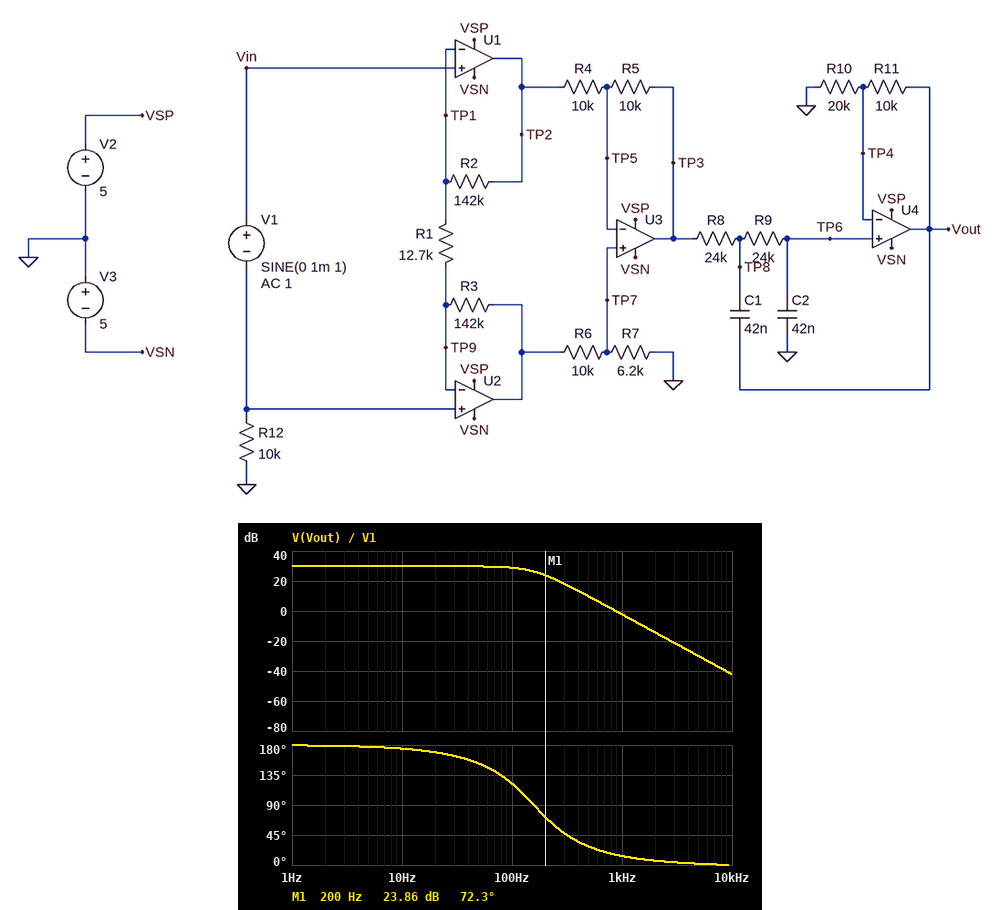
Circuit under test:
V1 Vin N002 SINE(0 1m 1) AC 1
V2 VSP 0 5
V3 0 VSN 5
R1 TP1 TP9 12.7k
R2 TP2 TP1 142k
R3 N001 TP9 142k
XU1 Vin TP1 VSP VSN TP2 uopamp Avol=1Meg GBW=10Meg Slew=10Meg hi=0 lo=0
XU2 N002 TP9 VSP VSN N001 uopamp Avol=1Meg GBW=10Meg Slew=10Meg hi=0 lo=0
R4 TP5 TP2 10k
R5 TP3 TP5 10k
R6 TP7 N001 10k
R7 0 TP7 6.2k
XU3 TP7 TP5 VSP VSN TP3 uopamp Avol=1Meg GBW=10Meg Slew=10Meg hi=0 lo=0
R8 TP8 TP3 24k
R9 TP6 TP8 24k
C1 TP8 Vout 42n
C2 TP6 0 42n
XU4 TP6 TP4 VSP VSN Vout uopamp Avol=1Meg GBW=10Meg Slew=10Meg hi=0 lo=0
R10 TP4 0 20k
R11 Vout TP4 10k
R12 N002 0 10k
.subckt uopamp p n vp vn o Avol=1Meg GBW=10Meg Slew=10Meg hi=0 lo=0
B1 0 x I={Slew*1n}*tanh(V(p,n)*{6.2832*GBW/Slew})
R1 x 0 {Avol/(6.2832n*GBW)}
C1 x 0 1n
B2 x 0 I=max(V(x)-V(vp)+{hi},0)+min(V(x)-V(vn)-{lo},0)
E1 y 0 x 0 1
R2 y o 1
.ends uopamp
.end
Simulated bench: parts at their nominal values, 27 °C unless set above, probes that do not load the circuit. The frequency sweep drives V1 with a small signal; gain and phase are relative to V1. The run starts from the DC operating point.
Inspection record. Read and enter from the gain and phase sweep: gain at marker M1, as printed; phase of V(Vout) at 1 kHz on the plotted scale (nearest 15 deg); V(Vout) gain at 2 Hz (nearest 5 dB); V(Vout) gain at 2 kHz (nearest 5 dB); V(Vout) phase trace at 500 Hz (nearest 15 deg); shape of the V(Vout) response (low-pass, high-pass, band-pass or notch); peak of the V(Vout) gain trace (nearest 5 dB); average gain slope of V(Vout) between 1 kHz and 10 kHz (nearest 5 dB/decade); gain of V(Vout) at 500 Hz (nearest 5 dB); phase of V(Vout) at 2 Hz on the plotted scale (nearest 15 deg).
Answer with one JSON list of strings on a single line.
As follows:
["23.86 dB", "15 deg", "30 dB", "-15 dB", "30 deg", "low-pass", "30 dB", "-40 dB/decade", "10 dB", "180 deg"]
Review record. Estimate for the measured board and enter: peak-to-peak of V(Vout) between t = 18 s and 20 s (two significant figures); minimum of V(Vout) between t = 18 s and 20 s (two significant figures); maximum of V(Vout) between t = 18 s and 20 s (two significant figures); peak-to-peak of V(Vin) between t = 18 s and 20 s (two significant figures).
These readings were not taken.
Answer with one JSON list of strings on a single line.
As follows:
["62 mV", "-31 mV", "31 mV", "2.0 mV"]
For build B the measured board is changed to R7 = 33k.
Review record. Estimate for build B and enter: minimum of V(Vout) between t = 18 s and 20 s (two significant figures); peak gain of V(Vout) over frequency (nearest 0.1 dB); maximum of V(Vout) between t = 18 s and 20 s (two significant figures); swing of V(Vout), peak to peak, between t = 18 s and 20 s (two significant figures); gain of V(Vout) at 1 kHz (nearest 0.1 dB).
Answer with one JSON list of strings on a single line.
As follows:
["-44 mV", "32.9 dB", "44 mV", "88 mV", "0.8 dB"]
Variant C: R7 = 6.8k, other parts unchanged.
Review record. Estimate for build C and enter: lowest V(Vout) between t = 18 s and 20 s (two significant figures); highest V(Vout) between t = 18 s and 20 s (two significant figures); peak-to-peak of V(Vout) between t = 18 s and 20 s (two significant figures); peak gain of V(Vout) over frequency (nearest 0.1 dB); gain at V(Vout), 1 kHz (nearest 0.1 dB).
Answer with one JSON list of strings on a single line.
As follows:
["-32 mV", "32 mV", "64 mV", "30.1 dB", "-2.0 dB"]
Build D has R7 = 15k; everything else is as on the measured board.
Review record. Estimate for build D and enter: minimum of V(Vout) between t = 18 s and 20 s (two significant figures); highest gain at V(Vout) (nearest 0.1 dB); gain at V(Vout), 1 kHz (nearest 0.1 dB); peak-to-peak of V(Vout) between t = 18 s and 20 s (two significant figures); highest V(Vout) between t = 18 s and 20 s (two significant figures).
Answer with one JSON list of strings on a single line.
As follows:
["-38 mV", "31.7 dB", "-0.4 dB", "77 mV", "38 mV"]
